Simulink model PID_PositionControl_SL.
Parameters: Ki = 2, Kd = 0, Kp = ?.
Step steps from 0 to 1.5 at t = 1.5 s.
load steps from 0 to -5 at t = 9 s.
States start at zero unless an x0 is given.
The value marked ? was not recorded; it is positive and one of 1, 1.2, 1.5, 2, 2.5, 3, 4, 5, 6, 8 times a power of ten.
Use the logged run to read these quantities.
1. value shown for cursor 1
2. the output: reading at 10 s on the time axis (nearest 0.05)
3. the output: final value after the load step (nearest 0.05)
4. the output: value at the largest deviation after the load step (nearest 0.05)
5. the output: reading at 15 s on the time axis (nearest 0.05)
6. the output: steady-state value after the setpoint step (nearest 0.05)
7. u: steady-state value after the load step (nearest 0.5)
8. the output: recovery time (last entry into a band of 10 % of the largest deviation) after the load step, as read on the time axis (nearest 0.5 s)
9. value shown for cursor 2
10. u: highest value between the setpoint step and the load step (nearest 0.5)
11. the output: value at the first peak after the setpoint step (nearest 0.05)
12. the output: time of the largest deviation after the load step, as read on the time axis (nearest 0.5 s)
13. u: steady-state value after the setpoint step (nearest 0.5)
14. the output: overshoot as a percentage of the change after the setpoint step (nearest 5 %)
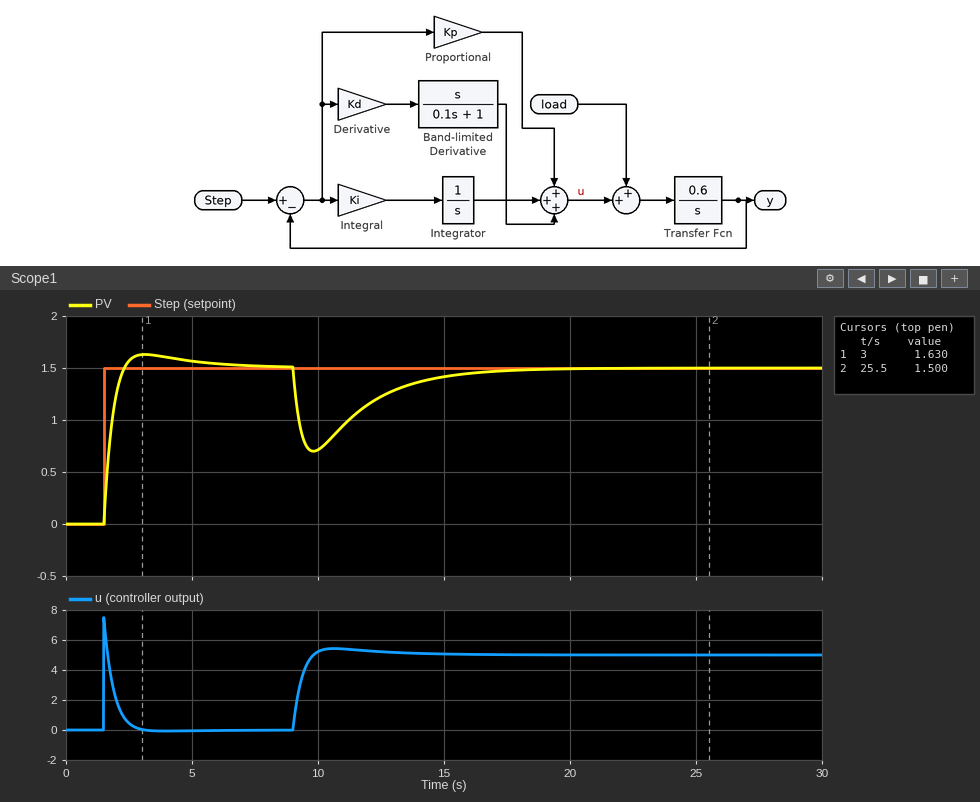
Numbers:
1.630
0.70
1.50
0.70
1.40
1.50
5.0
15.0 s
1.500
7.5
1.65
10.0 s
0.0
10 %
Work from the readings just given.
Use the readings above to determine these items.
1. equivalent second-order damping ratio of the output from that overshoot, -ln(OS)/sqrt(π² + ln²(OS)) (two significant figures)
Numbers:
0.59
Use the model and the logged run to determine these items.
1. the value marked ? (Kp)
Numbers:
5
